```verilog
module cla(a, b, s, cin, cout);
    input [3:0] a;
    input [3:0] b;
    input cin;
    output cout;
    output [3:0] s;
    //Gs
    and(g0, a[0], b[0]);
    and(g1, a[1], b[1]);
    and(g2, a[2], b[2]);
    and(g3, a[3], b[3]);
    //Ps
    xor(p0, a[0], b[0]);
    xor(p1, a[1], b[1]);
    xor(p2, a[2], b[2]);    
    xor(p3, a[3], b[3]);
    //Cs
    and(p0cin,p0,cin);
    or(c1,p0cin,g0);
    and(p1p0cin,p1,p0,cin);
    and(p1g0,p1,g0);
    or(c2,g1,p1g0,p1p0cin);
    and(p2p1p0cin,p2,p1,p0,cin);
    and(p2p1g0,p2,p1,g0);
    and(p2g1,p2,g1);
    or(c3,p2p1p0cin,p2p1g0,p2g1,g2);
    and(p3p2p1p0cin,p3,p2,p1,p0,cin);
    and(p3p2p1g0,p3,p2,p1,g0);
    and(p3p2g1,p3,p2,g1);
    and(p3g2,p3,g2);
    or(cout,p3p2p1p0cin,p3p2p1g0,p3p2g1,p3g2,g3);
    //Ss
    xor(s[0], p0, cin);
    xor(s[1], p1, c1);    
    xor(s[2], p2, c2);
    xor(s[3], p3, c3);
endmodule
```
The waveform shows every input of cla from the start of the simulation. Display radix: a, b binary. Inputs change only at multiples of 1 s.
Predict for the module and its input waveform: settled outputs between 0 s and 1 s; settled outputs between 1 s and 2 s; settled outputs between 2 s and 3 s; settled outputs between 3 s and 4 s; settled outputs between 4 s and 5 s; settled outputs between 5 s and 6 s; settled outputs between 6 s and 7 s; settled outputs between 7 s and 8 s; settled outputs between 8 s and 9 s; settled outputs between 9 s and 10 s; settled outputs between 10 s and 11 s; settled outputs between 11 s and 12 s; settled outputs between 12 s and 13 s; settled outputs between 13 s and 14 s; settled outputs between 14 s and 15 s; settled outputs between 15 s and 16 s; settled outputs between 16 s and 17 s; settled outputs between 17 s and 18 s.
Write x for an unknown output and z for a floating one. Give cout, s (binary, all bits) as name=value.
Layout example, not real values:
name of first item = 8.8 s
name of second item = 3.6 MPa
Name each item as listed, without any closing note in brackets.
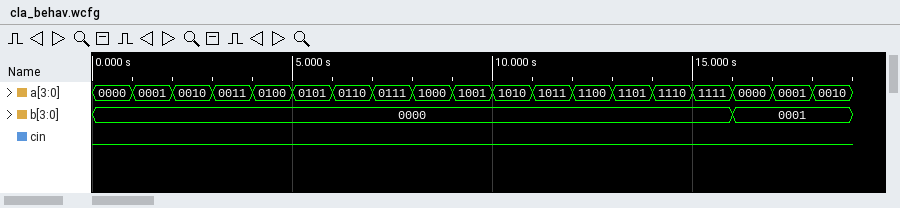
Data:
settled outputs between 0 s and 1 s = cout=0, s=0000
settled outputs between 1 s and 2 s = cout=0, s=0001
settled outputs between 2 s and 3 s = cout=0, s=0010
settled outputs between 3 s and 4 s = cout=0, s=0011
settled outputs between 4 s and 5 s = cout=0, s=0100
settled outputs between 5 s and 6 s = cout=0, s=0101
settled outputs between 6 s and 7 s = cout=0, s=0110
settled outputs between 7 s and 8 s = cout=0, s=0111
settled outputs between 8 s and 9 s = cout=0, s=1000
settled outputs between 9 s and 10 s = cout=0, s=1001
settled outputs between 10 s and 11 s = cout=0, s=1010
settled outputs between 11 s and 12 s = cout=0, s=1011
settled outputs between 12 s and 13 s = cout=0, s=1100
settled outputs between 13 s and 14 s = cout=0, s=1101
settled outputs between 14 s and 15 s = cout=0, s=1110
settled outputs between 15 s and 16 s = cout=0, s=1111
settled outputs between 16 s and 17 s = cout=0, s=0001
settled outputs between 17 s and 18 s = cout=0, s=0010
